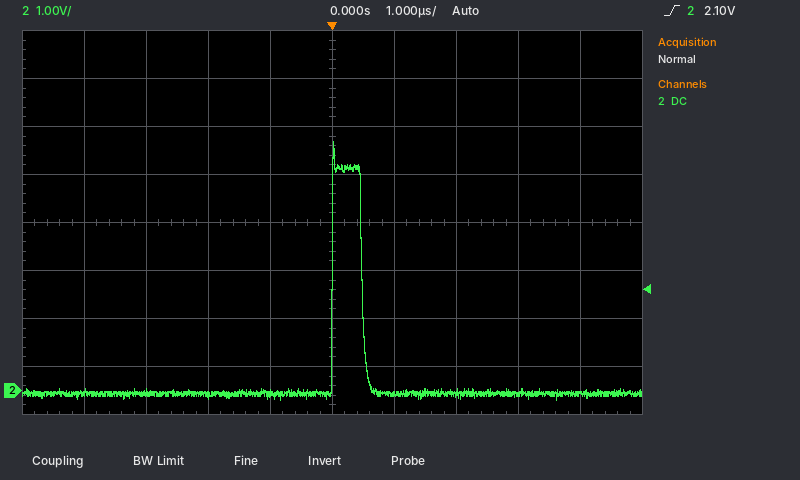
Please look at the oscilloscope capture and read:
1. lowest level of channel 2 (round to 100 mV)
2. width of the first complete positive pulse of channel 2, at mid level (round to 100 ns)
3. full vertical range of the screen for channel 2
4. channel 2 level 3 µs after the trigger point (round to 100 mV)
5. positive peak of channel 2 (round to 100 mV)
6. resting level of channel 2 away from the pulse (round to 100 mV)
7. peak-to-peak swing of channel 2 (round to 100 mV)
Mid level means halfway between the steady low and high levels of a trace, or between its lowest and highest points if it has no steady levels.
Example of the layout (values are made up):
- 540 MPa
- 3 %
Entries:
- -200 mV
- 500 ns
- 8 V
- -100 mV
- 5.2 V
- -100 mV
- 5.4 V
